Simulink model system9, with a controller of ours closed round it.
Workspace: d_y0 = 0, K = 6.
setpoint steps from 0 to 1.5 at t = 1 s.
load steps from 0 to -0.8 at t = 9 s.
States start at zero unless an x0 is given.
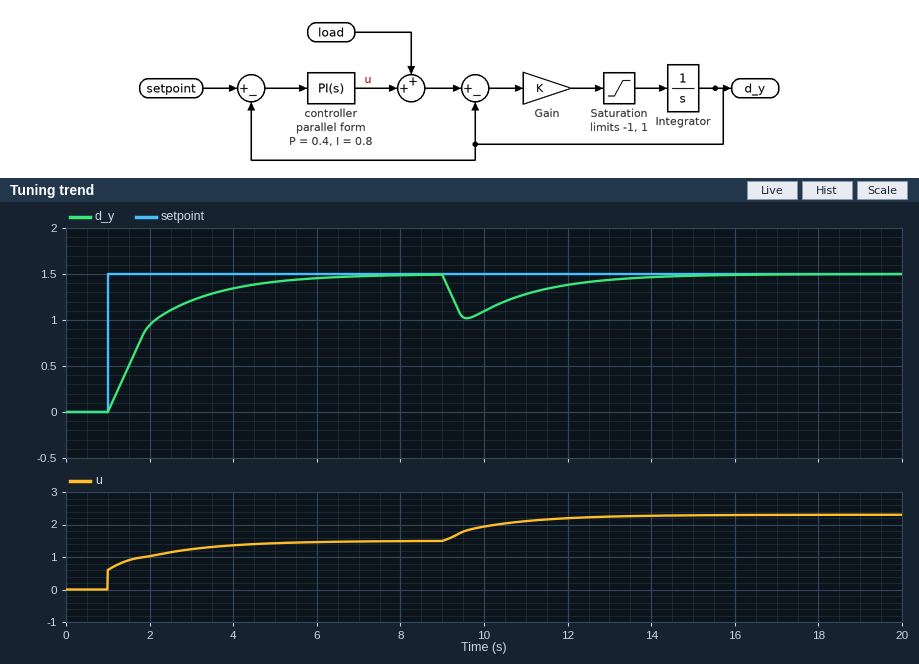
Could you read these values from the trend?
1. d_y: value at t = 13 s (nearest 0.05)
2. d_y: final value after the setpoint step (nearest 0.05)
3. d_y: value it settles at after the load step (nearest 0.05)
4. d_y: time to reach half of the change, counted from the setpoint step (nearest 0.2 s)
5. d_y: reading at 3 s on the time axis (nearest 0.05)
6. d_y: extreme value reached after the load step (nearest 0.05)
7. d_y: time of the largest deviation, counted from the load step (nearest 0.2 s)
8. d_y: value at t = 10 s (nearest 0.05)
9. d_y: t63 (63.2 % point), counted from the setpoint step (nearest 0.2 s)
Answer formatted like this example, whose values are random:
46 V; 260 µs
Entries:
1.45; 1.50; 1.50; 0.8 s; 1.20; 1.00; 0.6 s; 1.10; 1.0 s
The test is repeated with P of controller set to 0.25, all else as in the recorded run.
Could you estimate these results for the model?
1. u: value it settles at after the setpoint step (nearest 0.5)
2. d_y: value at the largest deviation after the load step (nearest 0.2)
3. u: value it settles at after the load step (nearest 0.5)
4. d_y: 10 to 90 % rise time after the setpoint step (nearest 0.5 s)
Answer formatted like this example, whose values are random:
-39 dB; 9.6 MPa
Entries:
1.5; 1.0; 2.5; 3.0 s
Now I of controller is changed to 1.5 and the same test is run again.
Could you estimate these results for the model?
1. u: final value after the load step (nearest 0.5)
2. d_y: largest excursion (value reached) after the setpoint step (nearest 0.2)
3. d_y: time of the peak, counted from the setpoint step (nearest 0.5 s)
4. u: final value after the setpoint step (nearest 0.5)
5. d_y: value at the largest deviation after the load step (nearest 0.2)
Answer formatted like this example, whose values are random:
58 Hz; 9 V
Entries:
2.5; 1.6; 2.0 s; 1.5; 1.0
